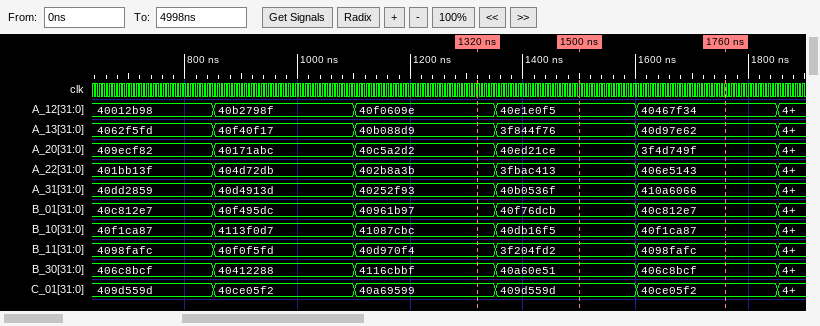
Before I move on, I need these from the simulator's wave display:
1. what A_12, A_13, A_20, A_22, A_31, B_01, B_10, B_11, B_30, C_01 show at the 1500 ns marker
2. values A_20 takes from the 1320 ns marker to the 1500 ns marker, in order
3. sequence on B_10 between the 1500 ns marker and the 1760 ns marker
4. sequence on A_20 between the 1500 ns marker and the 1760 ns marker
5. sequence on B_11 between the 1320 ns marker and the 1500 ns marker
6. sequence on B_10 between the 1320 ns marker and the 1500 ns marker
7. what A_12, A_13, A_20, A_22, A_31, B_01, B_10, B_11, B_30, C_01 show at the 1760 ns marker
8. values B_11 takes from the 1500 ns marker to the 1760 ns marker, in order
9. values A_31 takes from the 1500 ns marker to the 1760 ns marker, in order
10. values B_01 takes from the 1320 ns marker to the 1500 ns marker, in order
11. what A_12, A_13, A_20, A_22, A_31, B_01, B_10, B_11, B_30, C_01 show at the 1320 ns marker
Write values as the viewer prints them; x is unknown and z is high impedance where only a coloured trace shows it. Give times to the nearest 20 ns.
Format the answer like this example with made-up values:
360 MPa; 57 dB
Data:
A_12=40e1e0f5, A_13=3f844f76, A_20=40ed21ce, A_22=3fbac413, A_31=40b0536f, B_01=40f76dcb, B_10=40db16f5, B_11=3f204fd2, B_30=40a60e51, C_01=409d559d; 40c5a2d2, 40ed21ce; 40db16f5, 40f1ca87; 40ed21ce, 3f4d749f; 40d970f4, 3f204fd2; 41087cbc, 40db16f5; A_12=40467f34, A_13=40d97e62, A_20=3f4d749f, A_22=406e5143, A_31=410a6066, B_01=40c812e7, B_10=40f1ca87, B_11=4098fafc, B_30=406c8bcf, C_01=40ce05f2; 3f204fd2, 4098fafc; 40b0536f, 410a6066; 40961b97, 40f76dcb; A_12=40f0609e, A_13=40b088d9, A_20=40c5a2d2, A_22=402b8a3b, A_31=40252f93, B_01=40961b97, B_10=41087cbc, B_11=40d970f4, B_30=4116cbbf, C_01=40a69599
